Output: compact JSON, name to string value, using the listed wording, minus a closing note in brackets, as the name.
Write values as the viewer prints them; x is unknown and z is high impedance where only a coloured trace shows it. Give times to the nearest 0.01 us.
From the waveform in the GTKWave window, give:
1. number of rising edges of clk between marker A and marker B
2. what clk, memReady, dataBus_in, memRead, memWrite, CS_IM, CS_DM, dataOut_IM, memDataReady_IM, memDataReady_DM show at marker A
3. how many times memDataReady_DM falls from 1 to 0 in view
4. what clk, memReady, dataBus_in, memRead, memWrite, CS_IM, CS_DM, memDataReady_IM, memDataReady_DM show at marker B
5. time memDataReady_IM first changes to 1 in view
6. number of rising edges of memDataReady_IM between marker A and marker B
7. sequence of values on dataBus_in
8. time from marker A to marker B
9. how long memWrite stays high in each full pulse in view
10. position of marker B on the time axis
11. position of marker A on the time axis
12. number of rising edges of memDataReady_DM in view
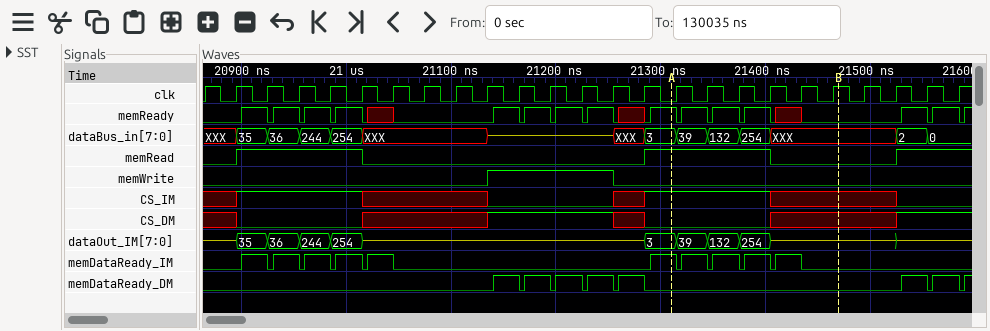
{"number of rising edges of clk between marker A and marker B": "6", "what clk, memReady, dataBus_in, memRead, memWrite, CS_IM, CS_DM, dataOut_IM, memDataReady_IM, memDataReady_DM show at marker A": "clk=0, memReady=1, dataBus_in=3, memRead=1, memWrite=0, CS_IM=1, CS_DM=0, dataOut_IM=3, memDataReady_IM=1, memDataReady_DM=0", "how many times memDataReady_DM falls from 1 to 0 in view": "7", "what clk, memReady, dataBus_in, memRead, memWrite, CS_IM, CS_DM, memDataReady_IM, memDataReady_DM show at marker B": "clk=1, memReady=0, dataBus_in=XXX, memRead=0, memWrite=0, CS_IM=x, CS_DM=x, memDataReady_IM=0, memDataReady_DM=0", "time memDataReady_IM first changes to 1 in view": "20.9 us", "number of rising edges of memDataReady_IM between marker A and marker B": "4", "sequence of values on dataBus_in": "XXX, 35, 36, 244, 254, XXX, z, XXX, 3, 39, 132, 254, XXX, 2, 0", "time from marker A to marker B": "0.16 us", "how long memWrite stays high in each full pulse in view": "0.12 us", "position of marker B on the time axis": "21.47 us", "position of marker A on the time axis": "21.31 us", "number of rising edges of memDataReady_DM in view": "8"}
